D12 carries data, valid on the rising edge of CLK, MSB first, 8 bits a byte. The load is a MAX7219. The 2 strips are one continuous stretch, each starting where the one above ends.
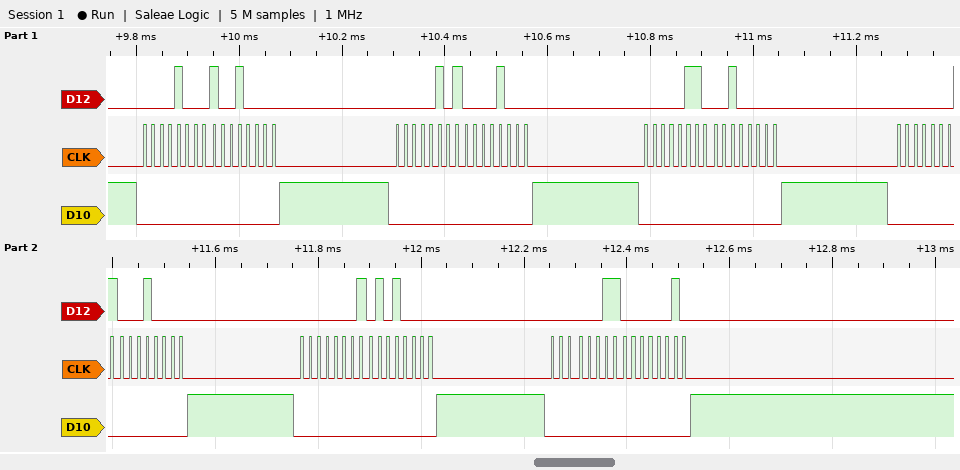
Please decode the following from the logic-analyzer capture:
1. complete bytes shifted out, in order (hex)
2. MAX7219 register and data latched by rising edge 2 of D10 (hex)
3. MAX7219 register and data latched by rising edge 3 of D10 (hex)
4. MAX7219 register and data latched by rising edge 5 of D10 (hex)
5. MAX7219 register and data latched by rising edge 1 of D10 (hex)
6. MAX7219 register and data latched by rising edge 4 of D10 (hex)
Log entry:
08 90 05 08 06 20 01 10 01 50 03 02
register 0x5, data 0x08
register 0x6, data 0x20
register 0x1, data 0x50
register 0x8, data 0x90
register 0x1, data 0x10
